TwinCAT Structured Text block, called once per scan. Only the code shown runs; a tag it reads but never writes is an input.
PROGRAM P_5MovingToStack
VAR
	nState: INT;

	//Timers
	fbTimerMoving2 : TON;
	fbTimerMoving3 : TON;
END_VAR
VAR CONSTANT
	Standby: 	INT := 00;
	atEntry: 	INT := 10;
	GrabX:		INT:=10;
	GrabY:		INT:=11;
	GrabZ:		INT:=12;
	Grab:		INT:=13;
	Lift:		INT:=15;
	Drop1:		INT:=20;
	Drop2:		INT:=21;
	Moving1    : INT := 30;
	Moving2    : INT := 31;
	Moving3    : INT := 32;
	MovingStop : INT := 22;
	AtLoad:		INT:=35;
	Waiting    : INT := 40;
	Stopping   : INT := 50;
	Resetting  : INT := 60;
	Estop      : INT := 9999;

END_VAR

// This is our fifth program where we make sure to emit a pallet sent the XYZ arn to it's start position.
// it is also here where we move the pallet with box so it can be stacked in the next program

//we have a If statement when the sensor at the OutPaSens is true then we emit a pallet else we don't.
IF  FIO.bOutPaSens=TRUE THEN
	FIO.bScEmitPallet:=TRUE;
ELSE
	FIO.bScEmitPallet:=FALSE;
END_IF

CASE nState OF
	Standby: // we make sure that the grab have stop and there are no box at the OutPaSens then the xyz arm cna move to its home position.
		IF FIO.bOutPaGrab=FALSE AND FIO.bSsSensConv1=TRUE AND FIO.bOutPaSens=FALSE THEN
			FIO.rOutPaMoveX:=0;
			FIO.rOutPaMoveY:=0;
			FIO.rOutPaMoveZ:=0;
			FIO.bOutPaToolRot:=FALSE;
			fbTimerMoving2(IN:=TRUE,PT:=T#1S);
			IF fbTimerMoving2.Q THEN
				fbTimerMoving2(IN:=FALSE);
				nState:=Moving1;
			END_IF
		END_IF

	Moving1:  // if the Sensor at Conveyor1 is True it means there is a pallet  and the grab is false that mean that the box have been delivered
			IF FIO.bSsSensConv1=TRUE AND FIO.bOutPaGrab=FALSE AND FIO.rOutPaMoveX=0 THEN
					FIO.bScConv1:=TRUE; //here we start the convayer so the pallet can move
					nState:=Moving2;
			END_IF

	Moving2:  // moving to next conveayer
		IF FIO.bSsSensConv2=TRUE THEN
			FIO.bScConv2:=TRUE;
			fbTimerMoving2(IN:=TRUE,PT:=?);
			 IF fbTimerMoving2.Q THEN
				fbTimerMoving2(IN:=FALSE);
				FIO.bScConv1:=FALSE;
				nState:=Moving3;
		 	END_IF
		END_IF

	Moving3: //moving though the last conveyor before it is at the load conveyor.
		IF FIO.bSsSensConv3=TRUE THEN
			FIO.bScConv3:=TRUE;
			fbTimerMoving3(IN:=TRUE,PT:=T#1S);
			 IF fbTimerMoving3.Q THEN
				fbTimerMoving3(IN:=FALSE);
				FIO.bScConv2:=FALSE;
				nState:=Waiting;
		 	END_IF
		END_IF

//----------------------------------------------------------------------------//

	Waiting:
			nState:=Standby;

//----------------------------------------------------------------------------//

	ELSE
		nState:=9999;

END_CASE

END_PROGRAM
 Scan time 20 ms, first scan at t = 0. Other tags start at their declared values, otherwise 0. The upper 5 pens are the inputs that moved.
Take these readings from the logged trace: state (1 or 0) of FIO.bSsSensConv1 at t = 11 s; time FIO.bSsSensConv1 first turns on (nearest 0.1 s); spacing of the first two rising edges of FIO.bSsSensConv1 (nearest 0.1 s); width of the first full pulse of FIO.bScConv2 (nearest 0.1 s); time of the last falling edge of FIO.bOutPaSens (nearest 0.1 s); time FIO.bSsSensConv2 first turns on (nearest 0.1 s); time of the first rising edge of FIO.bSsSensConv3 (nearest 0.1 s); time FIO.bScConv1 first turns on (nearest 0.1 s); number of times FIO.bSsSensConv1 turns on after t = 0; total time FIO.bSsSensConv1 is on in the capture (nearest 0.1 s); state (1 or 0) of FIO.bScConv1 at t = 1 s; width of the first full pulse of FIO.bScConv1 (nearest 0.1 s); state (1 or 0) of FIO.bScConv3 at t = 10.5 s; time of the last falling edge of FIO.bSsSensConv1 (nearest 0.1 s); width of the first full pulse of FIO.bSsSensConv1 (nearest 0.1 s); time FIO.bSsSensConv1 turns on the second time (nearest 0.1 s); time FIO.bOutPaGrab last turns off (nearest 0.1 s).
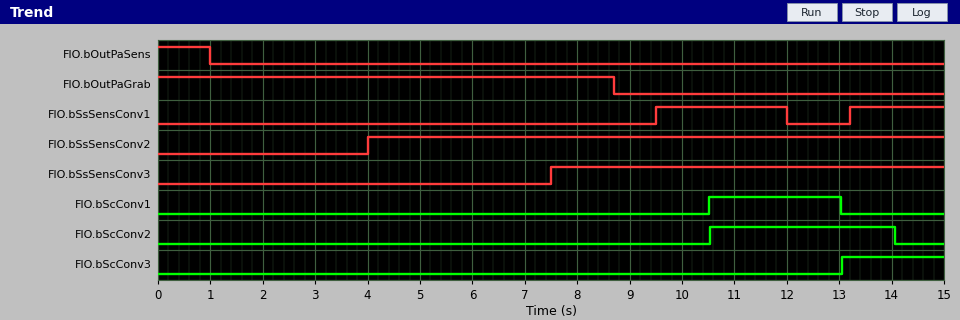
1
9.5 s
3.7 s
3.5 s
1.0 s
4.0 s
7.5 s
10.5 s
2
4.3 s
0
2.5 s
0
12.0 s
2.5 s
13.2 s
8.7 s
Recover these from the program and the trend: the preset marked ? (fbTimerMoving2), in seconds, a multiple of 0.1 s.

2.5 s
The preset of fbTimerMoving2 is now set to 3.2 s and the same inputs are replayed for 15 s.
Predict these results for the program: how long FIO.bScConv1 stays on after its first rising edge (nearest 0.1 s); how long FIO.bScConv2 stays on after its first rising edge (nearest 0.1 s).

3.2 s
4.2 s
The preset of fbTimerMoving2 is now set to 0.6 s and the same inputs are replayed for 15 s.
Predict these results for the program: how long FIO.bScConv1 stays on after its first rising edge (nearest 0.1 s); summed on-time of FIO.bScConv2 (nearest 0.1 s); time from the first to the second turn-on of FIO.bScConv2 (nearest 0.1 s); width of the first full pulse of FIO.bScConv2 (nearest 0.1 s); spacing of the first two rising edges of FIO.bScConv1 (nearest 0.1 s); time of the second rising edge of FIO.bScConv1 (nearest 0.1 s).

0.6 s
2.4 s
3.7 s
1.6 s
3.7 s
14.2 s
